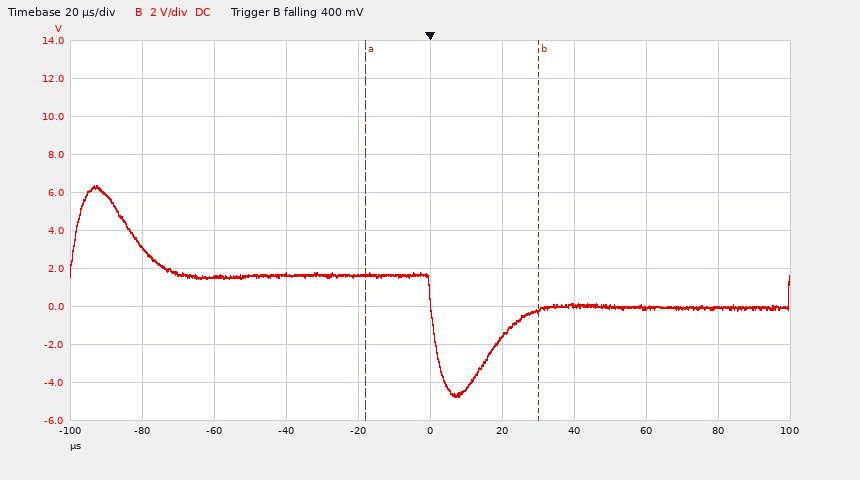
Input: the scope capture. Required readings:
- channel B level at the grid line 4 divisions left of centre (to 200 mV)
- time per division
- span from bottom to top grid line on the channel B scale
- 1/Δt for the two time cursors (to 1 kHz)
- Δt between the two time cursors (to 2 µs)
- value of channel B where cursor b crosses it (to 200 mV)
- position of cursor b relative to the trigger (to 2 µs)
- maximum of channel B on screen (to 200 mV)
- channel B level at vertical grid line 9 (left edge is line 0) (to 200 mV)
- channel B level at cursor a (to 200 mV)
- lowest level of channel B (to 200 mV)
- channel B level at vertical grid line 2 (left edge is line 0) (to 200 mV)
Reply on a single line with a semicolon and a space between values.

3.2 V; 20 µs; 20 V; 21 kHz; 48 µs; -200 mV; +30 µs; 6.4 V; 0.0 V; 1.6 V; -4.8 V; 1.6 V
